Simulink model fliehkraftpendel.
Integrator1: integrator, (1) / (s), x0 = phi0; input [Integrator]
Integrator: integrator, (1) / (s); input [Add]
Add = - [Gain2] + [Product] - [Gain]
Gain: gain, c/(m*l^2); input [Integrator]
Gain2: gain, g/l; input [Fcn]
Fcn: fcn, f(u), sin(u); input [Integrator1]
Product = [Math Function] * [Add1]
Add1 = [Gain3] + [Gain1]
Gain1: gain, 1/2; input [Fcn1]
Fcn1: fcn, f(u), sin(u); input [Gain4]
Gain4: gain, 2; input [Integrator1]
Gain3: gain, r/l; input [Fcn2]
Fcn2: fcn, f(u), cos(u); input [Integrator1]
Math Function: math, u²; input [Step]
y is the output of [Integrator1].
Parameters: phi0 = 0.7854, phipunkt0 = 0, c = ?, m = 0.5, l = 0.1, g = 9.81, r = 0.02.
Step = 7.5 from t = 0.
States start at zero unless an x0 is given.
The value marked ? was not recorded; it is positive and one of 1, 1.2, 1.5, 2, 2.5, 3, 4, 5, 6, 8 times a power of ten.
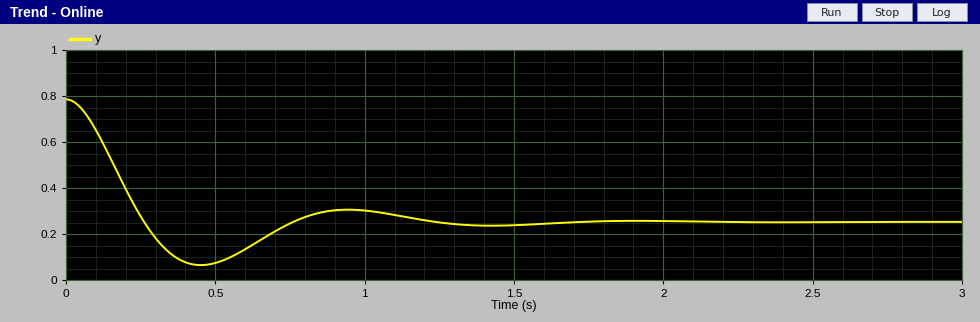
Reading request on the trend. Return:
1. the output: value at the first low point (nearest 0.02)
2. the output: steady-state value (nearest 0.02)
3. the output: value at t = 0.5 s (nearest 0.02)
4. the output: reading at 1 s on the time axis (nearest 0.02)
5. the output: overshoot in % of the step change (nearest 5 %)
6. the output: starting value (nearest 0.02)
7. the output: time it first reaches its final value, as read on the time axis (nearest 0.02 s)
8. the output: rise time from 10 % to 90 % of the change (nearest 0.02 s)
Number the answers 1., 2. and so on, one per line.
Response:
1. 0.06
2. 0.26
3. 0.08
4. 0.30
5. 35 %
6. 0.78
7. 0.26 s
8. 0.18 s
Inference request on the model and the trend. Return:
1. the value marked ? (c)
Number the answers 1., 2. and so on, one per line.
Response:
1. 0.025
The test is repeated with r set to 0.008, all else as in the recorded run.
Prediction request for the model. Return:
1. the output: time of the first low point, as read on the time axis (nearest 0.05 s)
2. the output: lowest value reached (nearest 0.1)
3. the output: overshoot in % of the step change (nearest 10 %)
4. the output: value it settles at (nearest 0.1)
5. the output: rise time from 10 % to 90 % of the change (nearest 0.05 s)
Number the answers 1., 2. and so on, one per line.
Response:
1. 0.50 s
2. -0.1
3. 30 %
4. 0.1
5. 0.20 s
